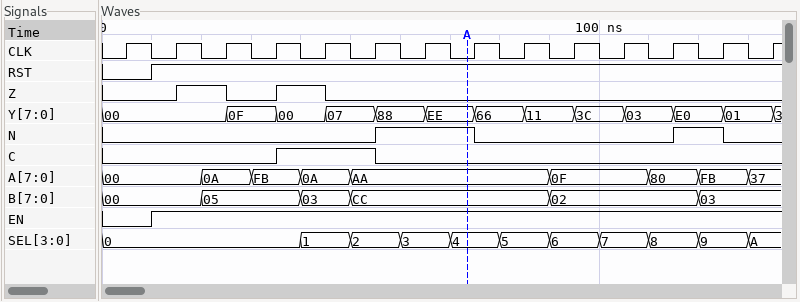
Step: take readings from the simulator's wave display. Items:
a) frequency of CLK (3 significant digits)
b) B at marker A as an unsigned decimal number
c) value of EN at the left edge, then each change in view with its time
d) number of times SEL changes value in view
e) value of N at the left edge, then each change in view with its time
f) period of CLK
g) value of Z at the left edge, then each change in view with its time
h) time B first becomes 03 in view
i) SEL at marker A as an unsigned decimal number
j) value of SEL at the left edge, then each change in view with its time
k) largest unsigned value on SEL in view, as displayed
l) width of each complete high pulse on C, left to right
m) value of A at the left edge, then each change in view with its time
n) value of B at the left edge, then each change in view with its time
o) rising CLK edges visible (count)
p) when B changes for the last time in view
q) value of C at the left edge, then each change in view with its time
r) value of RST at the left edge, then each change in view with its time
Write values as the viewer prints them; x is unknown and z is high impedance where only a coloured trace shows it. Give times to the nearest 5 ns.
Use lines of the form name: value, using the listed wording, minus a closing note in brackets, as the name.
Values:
frequency of CLK: 100 MHz
B at marker A as an unsigned decimal number: 204
value of EN at the left edge, then each change in view with its time: 0, 1 at 10 ns
number of times SEL changes value in view: 10
value of N at the left edge, then each change in view with its time: 0, 1 at 55 ns, 0 at 75 ns, 1 at 115 ns, 0 at 125 ns
period of CLK: 10 ns
value of Z at the left edge, then each change in view with its time: 0, 1 at 15 ns, 0 at 25 ns, 1 at 35 ns, 0 at 45 ns
time B first becomes 03 in view: 40 ns
SEL at marker A as an unsigned decimal number: 4
value of SEL at the left edge, then each change in view with its time: 0, 1 at 40 ns, 2 at 50 ns, 3 at 60 ns, 4 at 70 ns, 5 at 80 ns, 6 at 90 ns, 7 at 100 ns, 8 at 110 ns, 9 at 120 ns, A at 130 ns
largest unsigned value on SEL in view, as displayed: A
width of each complete high pulse on C, left to right: 20 ns
value of A at the left edge, then each change in view with its time: 00, 0A at 20 ns, FB at 30 ns, 0A at 40 ns, AA at 50 ns, 0F at 90 ns, 80 at 110 ns, FB at 120 ns, 37 at 130 ns
value of B at the left edge, then each change in view with its time: 00, 05 at 20 ns, 03 at 40 ns, CC at 50 ns, 02 at 90 ns, 03 at 120 ns
rising CLK edges visible: 14
when B changes for the last time in view: 120 ns
value of C at the left edge, then each change in view with its time: 0, 1 at 35 ns, 0 at 55 ns
value of RST at the left edge, then each change in view with its time: 0, 1 at 10 ns
